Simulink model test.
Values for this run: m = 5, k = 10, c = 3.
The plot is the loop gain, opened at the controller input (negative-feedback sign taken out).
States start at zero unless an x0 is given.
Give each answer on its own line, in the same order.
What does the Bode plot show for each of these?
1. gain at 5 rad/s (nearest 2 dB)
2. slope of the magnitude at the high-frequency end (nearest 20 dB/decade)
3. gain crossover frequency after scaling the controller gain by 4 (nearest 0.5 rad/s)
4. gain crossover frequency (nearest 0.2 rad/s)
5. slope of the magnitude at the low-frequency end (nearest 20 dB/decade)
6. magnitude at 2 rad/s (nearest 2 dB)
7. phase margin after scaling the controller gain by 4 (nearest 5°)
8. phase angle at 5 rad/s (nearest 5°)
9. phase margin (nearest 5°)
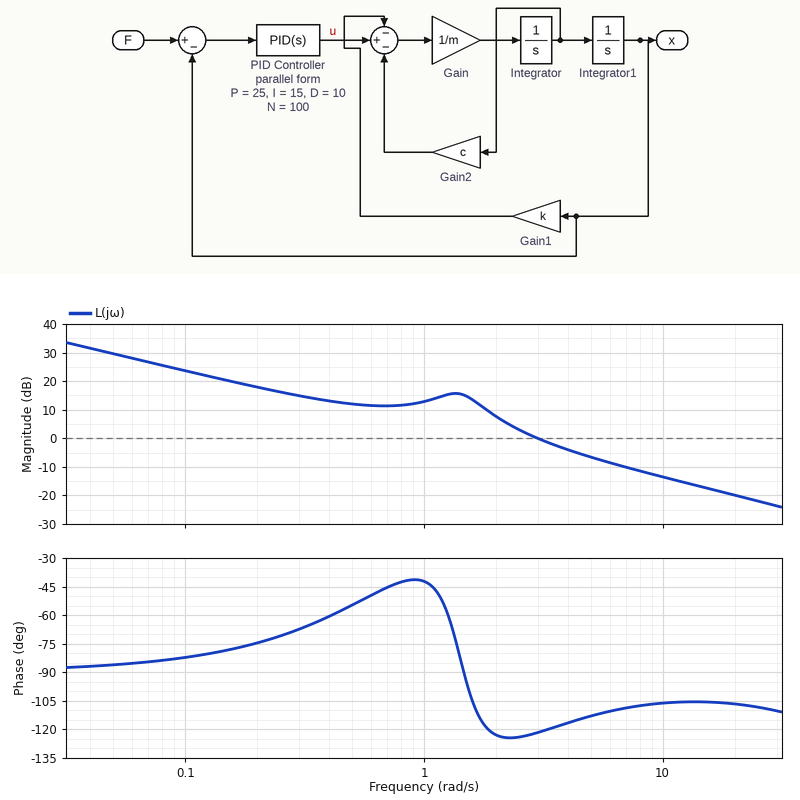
-6 dB
-20 dB/decade
8.5 rad/s
3.0 rad/s
-20 dB/decade
8 dB
75°
-115°
60°
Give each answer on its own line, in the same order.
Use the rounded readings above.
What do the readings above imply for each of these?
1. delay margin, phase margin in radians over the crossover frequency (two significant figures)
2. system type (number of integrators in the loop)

0.35 s
1
